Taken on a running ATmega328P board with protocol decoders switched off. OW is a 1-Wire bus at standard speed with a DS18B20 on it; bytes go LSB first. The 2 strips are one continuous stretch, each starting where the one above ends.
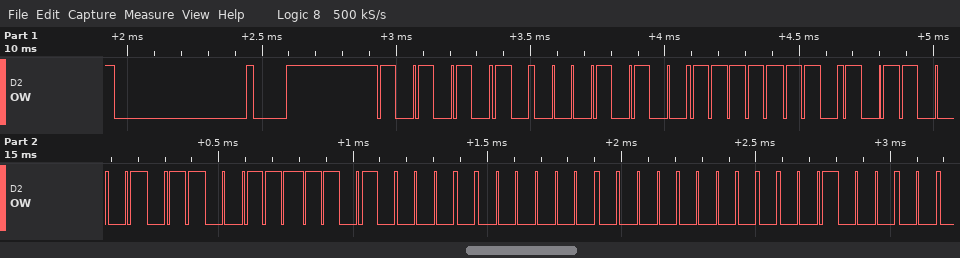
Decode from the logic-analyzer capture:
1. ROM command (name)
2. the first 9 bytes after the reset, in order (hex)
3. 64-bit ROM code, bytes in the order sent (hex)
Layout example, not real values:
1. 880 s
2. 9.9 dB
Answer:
1. Match ROM
2. 55 28 7F 8D E6 0B 00 00 04
3. 28 7F 8D E6 0B 00 00 04
